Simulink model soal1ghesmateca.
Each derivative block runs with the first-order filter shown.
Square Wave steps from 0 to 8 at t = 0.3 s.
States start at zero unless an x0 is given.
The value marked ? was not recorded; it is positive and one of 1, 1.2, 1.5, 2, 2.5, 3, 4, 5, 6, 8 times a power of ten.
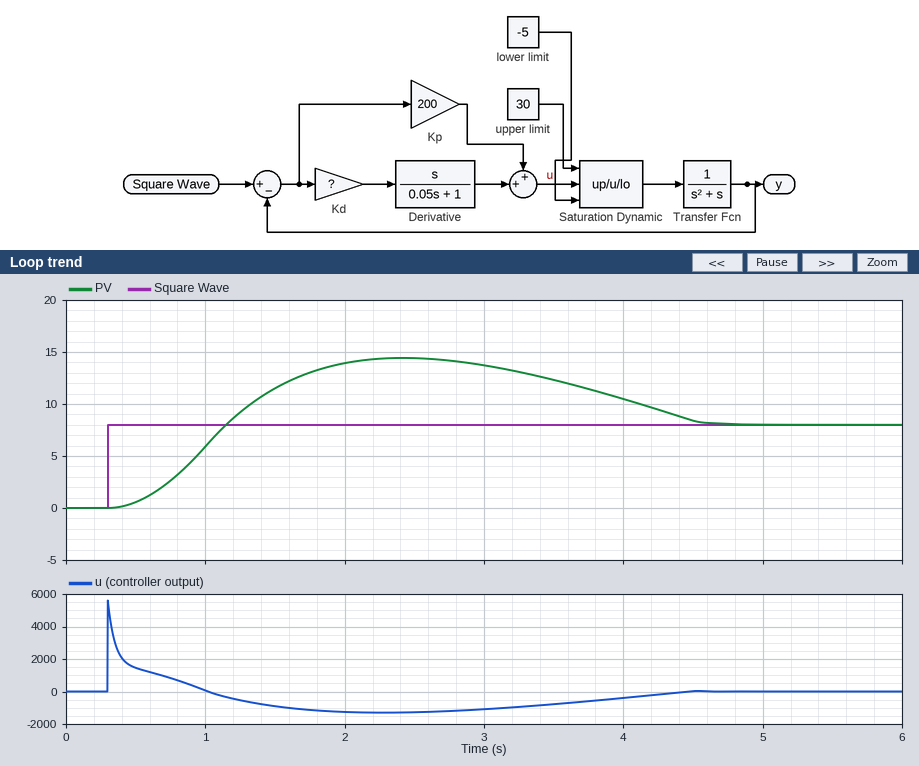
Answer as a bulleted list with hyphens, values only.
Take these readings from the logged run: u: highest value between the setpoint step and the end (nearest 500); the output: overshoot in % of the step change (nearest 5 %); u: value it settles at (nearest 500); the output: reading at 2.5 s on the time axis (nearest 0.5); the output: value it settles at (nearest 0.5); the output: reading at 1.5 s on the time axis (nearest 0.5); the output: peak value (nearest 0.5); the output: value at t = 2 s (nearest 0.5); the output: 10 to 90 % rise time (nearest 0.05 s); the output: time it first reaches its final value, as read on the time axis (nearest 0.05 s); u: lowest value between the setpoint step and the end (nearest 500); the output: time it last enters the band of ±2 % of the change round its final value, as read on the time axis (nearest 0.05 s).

- 5500
- 80 %
- 0
- 14.5
- 8.0
- 11.5
- 14.5
- 14.0
- 0.55 s
- 1.15 s
- -1500
- 4.65 s
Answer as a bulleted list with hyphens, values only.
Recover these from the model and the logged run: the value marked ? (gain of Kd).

- 25
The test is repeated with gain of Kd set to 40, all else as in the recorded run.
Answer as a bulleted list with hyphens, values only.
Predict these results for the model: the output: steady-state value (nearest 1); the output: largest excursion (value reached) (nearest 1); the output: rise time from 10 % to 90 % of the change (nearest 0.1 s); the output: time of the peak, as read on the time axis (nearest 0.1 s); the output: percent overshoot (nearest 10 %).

- 8
- 13
- 0.6 s
- 2.3 s
- 60 %
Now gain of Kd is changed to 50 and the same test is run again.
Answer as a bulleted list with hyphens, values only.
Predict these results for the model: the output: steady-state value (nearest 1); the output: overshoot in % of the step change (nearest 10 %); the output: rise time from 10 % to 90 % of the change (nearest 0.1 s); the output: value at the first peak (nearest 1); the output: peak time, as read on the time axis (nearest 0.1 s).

- 8
- 50 %
- 0.6 s
- 12
- 2.2 s
